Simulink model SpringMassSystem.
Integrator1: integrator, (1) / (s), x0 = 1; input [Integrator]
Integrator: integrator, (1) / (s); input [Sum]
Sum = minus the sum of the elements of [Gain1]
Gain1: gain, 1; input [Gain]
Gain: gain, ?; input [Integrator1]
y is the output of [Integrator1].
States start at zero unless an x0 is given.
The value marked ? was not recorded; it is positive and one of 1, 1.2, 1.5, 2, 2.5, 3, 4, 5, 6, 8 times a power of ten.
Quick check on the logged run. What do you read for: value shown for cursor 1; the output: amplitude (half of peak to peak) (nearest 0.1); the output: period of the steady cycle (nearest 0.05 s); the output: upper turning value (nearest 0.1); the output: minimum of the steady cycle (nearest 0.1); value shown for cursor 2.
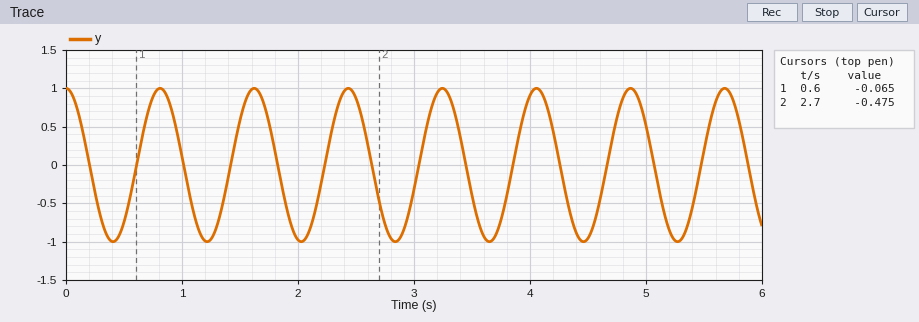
-0.065
1.0
0.80 s
1.0
-1.0
-0.475
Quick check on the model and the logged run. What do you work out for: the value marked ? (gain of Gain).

60
